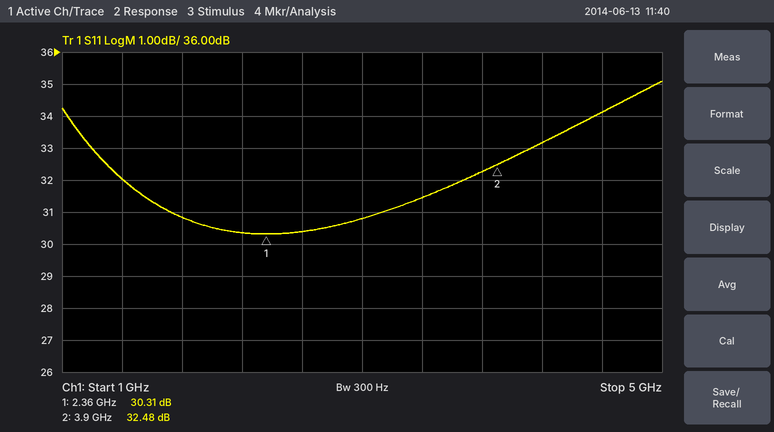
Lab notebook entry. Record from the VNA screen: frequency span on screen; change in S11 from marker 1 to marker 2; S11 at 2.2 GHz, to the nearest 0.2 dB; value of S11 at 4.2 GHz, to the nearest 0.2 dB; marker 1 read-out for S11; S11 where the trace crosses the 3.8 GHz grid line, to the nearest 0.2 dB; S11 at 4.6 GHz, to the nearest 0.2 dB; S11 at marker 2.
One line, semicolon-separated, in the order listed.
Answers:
4 GHz; 2.17 dB; 30.4 dB; 33.2 dB; 30.31 dB; 32.2 dB; 34.2 dB; 32.48 dB
